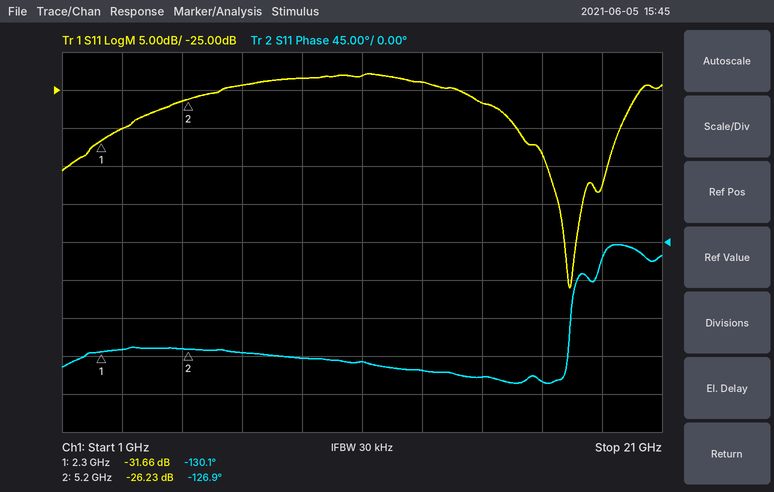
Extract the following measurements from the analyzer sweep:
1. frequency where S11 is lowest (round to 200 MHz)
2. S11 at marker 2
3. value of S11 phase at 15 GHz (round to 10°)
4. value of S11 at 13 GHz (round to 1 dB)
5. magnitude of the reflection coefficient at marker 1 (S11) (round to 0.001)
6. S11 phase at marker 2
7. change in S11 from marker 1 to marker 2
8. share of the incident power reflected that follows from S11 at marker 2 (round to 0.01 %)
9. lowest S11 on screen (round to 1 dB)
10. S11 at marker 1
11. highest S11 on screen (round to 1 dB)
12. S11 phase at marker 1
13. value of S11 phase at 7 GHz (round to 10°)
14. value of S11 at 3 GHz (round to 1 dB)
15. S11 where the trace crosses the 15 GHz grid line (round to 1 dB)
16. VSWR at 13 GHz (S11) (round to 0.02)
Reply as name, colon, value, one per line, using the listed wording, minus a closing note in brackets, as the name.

frequency where S11 is lowest: 18.0 GHz
S11 at marker 2: -26.23 dB
value of S11 phase at 15 GHz: -160°
value of S11 at 13 GHz: -24 dB
magnitude of the reflection coefficient at marker 1 (S11): 0.026
S11 phase at marker 2: -126.9°
change in S11 from marker 1 to marker 2: 5.43 dB
share of the incident power reflected that follows from S11 at marker 2: 0.24 %
lowest S11 on screen: -51 dB
S11 at marker 1: -31.66 dB
highest S11 on screen: -23 dB
S11 phase at marker 1: -130.1°
value of S11 phase at 7 GHz: -130°
value of S11 at 3 GHz: -30 dB
S11 where the trace crosses the 15 GHz grid line: -27 dB
VSWR at 13 GHz (S11): 1.14
